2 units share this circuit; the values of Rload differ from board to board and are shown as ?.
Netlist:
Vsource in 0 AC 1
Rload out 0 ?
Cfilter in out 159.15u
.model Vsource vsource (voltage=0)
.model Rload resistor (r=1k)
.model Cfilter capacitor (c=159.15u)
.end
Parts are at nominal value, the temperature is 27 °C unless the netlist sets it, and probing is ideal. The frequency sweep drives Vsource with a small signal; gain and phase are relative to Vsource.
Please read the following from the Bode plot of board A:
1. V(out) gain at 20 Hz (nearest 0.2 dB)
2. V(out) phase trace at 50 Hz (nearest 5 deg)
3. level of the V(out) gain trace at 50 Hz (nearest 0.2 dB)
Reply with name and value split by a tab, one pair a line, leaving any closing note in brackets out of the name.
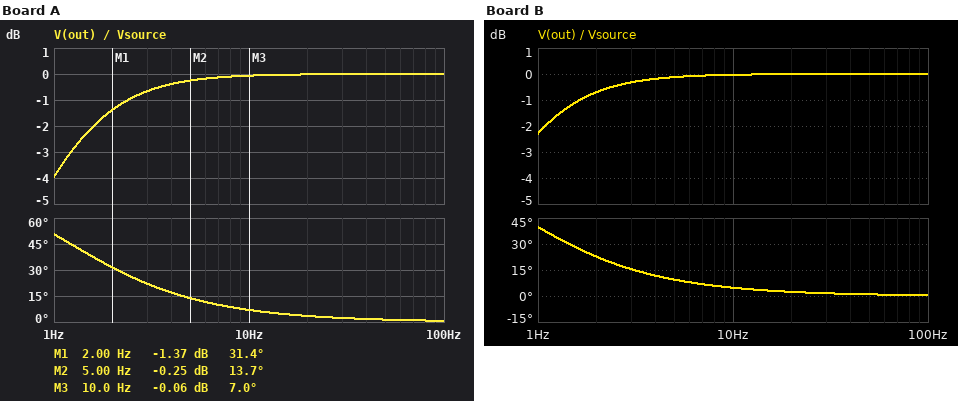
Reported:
V(out) gain at 20 Hz	0 dB
V(out) phase trace at 50 Hz	0 deg
level of the V(out) gain trace at 50 Hz	0 dB
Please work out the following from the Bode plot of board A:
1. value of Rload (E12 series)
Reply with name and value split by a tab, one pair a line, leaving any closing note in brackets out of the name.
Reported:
value of Rload	820 Ω
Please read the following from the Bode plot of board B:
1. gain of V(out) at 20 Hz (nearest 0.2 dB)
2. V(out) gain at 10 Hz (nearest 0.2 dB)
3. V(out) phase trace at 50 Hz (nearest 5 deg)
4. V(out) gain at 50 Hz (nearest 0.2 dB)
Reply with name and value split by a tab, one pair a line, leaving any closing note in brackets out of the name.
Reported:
gain of V(out) at 20 Hz	0 dB
V(out) gain at 10 Hz	0 dB
V(out) phase trace at 50 Hz	0 deg
V(out) gain at 50 Hz	0 dB
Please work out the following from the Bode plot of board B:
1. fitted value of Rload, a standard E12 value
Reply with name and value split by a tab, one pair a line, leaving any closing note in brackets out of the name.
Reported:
fitted value of Rload, a standard E12 value	1.2 kΩ
